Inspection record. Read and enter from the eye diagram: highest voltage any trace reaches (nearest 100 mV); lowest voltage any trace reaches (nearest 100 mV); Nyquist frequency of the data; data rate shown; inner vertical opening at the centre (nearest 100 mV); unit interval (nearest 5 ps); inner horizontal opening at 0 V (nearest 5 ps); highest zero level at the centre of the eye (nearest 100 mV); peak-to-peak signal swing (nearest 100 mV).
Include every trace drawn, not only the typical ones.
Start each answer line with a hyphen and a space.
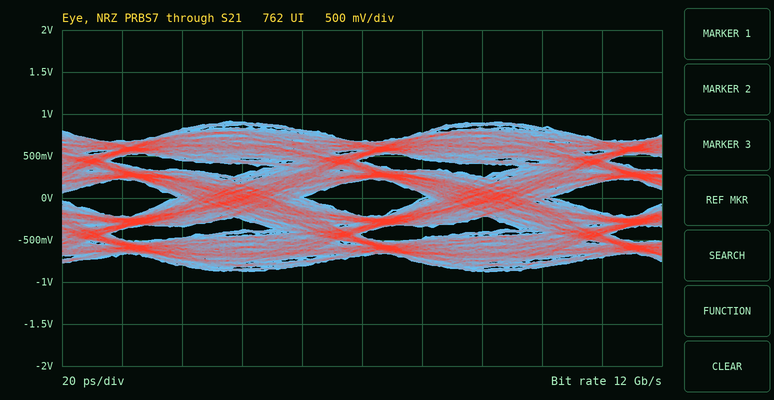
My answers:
- 900 mV
- -900 mV
- 6 GHz
- 12 Gb/s
- 400 mV
- 85 ps
- 40 ps
- -200 mV
- 1.8 V
